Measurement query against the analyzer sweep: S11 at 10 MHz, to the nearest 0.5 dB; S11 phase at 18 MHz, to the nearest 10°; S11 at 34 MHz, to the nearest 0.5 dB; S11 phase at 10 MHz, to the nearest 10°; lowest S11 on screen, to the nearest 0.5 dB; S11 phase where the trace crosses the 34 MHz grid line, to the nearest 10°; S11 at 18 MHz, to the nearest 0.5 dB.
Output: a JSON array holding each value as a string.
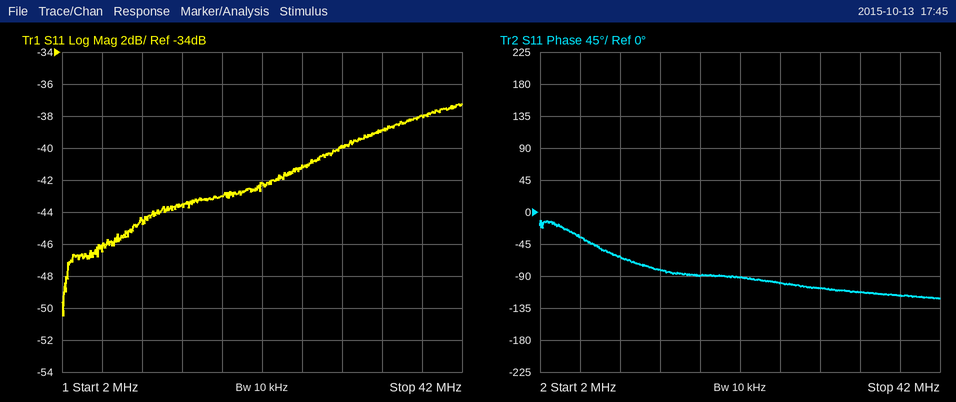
["-44.5 dB", "-90°", "-39.0 dB", "-60°", "-50.5 dB", "-110°", "-43.0 dB"]
